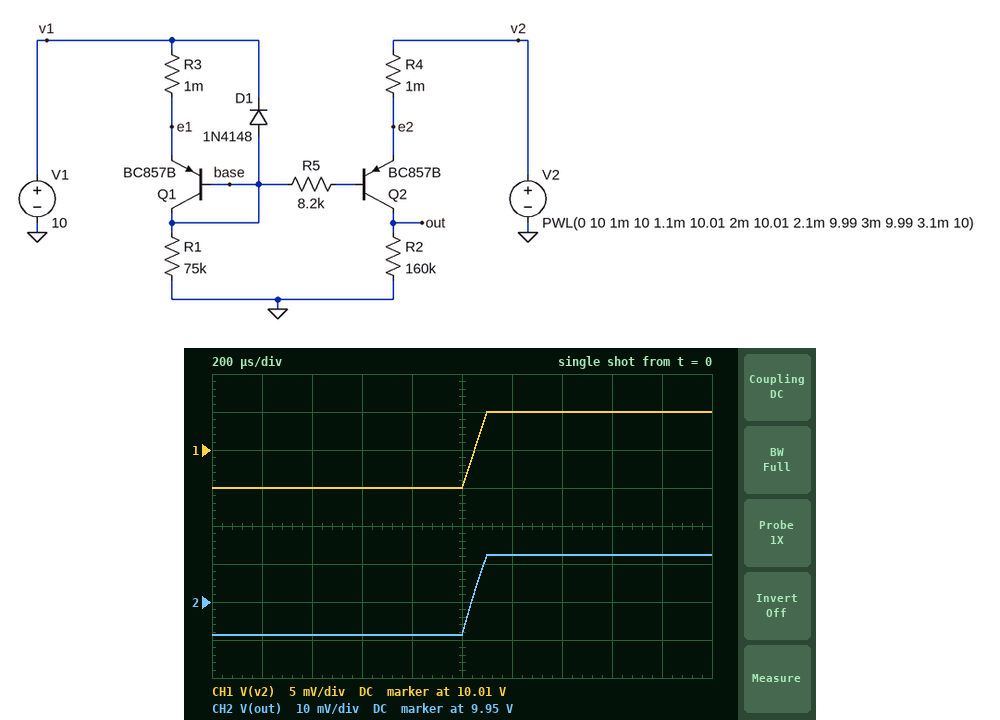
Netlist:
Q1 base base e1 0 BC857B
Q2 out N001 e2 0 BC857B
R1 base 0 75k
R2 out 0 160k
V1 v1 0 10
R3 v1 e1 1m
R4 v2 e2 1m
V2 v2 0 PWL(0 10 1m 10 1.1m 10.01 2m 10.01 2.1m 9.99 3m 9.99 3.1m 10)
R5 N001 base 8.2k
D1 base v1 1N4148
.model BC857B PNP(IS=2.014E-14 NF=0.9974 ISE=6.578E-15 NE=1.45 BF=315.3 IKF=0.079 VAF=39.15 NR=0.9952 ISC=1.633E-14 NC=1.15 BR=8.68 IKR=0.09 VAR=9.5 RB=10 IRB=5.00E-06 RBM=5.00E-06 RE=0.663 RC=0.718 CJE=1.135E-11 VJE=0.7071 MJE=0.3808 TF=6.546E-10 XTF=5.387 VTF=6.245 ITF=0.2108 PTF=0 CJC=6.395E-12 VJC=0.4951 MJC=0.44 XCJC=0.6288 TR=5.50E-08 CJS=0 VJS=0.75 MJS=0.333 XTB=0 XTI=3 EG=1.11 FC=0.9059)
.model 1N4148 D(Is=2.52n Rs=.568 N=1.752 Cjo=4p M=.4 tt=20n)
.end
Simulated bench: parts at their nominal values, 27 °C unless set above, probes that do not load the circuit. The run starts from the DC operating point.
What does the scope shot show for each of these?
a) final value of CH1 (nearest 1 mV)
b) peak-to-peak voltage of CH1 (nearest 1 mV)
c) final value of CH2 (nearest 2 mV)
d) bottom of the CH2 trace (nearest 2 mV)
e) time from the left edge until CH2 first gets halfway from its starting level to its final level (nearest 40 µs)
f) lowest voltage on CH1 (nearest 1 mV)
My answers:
10.010 V
10 mV
9.962 V
9.942 V
1.04 ms
10.000 V
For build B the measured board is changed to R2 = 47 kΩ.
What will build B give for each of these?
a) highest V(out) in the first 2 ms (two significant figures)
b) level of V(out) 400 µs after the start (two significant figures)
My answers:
7.6 V
5.7 V
